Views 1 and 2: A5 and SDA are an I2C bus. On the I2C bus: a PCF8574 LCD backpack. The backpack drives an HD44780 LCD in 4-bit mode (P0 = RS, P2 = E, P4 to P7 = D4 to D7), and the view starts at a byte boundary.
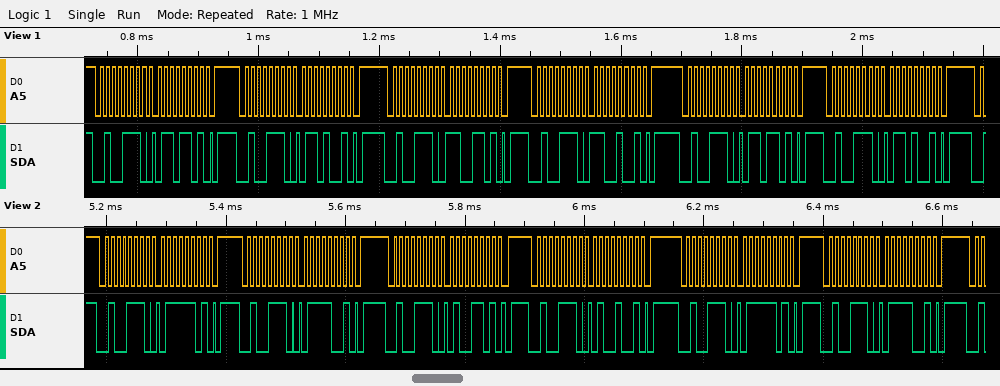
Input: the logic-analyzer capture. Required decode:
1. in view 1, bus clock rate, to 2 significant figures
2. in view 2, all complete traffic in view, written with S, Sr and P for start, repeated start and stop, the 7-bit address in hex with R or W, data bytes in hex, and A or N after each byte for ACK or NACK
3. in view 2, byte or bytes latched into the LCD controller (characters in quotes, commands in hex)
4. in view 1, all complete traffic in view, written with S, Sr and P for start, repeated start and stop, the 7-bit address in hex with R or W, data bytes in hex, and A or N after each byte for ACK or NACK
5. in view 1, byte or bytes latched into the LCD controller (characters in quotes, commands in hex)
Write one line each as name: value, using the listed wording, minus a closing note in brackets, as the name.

in view 1, bus clock rate, to 2 significant figures: 100 kHz
in view 2, all complete traffic in view, written with S, Sr and P for start, repeated start and stop, the 7-bit address in hex with R or W, data bytes in hex, and A or N after each byte for ACK or NACK: S 27W A 7D A P S 27W A 79 A P S 27W A 4D A P S 27W A 49 A P S 27W A 7D A P S 27W A 79 A P
in view 2, byte or bytes latched into the LCD controller: 't'
in view 1, all complete traffic in view, written with S, Sr and P for start, repeated start and stop, the 7-bit address in hex with R or W, data bytes in hex, and A or N after each byte for ACK or NACK: S 27W A 6D A P S 27W A 69 A P S 27W A CD A P S 27W A C9 A P S 27W A 6D A P S 27W A 69 A P
in view 1, byte or bytes latched into the LCD controller: 'l'
